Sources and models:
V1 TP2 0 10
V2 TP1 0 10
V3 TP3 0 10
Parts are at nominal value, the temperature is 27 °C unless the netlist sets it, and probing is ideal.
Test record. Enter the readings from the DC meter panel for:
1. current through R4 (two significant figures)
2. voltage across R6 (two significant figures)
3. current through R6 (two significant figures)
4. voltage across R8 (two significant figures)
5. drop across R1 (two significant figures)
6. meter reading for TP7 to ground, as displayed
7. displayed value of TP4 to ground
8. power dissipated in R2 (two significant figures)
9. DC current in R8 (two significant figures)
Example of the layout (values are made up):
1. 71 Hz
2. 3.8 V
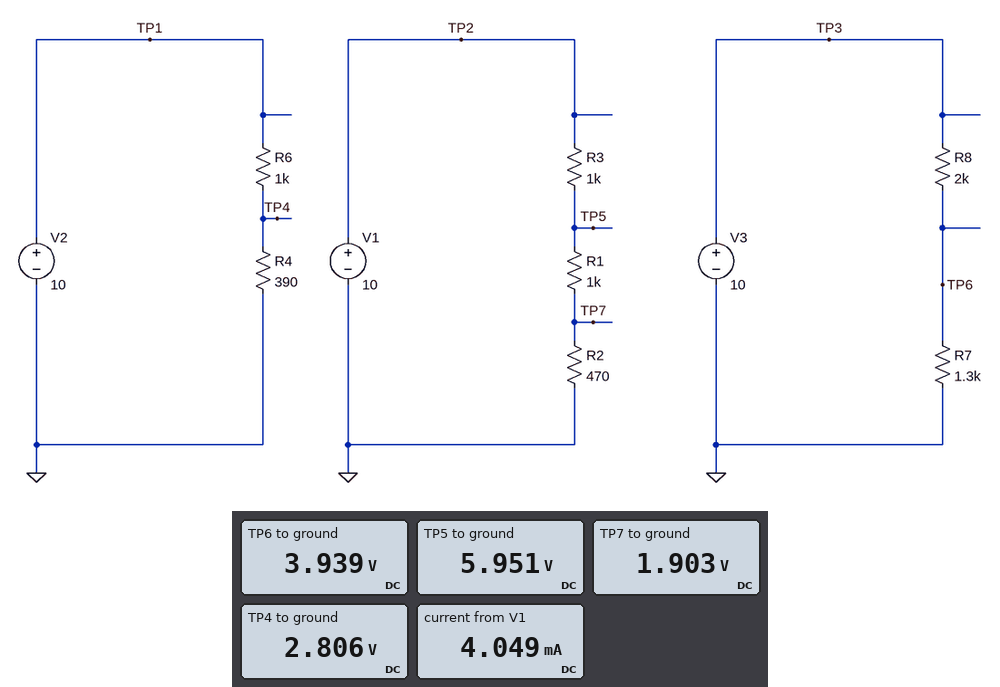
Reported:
1. 7.2 mA
2. 7.2 V
3. 7.2 mA
4. 6.1 V
5. 4.0 V
6. 1.903 V
7. 2.806 V
8. 7.7 mW
9. 3.0 mA
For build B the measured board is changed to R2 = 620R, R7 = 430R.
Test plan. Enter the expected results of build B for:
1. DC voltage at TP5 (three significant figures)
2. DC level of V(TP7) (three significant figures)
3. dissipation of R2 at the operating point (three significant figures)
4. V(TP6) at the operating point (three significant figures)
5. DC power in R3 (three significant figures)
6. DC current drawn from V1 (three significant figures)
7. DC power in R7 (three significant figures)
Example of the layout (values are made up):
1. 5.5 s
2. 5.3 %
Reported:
1. 6.18 V
2. 2.37 V
3. 9.03 mW
4. 1.77 V
5. 14.6 mW
6. 3.82 mA
7. 7.28 mW
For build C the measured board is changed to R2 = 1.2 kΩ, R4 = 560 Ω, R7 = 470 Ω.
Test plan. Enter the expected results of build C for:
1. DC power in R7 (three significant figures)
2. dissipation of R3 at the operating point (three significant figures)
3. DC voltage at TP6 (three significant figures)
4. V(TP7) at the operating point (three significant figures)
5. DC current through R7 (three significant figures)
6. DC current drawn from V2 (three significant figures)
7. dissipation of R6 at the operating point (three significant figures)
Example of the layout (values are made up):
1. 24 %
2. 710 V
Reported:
1. 7.70 mW
2. 9.77 mW
3. 1.90 V
4. 3.75 V
5. 4.05 mA
6. 6.41 mA
7. 41.1 mW
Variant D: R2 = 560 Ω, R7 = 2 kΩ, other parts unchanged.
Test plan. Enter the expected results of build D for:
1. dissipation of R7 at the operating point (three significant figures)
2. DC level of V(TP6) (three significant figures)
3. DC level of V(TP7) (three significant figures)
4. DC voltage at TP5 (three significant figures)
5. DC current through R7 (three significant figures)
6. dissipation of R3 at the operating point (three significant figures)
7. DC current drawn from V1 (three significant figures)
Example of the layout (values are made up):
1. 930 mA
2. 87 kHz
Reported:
1. 12.5 mW
2. 5.00 V
3. 2.19 V
4. 6.09 V
5. 2.50 mA
6. 15.3 mW
7. 3.91 mA
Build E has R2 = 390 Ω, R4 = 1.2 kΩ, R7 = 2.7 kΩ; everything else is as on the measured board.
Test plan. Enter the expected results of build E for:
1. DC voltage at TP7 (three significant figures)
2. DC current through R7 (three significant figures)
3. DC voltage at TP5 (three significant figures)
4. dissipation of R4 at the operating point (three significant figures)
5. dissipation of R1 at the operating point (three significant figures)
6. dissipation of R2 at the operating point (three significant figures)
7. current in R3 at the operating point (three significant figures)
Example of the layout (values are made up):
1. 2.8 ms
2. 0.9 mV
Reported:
1. 1.63 V
2. 2.13 mA
3. 5.82 V
4. 24.8 mW
5. 17.5 mW
6. 6.83 mW
7. 4.18 mA
